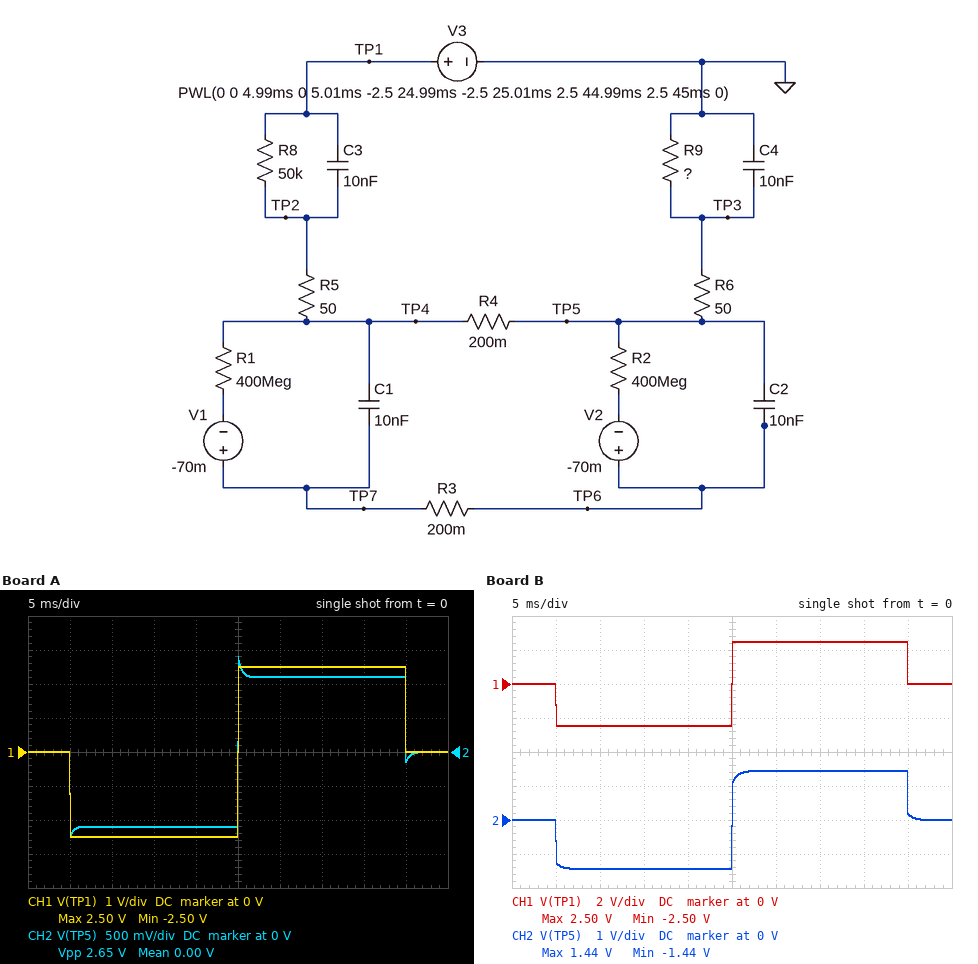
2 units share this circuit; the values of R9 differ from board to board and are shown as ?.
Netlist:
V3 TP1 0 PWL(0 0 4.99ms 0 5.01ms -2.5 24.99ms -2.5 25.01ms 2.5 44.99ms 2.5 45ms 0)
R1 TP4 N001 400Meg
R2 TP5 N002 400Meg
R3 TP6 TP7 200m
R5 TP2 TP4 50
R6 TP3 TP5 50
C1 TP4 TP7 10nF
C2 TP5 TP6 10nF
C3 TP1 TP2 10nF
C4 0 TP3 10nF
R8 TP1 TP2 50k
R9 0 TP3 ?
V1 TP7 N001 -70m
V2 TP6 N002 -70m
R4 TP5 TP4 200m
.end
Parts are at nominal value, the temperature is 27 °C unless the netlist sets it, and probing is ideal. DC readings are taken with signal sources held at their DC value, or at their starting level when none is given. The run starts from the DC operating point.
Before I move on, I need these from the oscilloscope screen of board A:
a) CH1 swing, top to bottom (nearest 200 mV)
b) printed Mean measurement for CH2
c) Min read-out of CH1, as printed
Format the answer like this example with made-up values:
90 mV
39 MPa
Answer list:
5.0 V
0.00 V
-2.50 V
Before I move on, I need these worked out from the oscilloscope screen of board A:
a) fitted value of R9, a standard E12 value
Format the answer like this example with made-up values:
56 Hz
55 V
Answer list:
39 kΩ
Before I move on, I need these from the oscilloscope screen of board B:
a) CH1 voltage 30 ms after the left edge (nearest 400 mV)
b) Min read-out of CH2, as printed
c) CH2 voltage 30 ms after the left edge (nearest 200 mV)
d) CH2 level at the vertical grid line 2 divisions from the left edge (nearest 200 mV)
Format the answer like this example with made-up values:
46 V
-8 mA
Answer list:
2.4 V
-1.44 V
1.4 V
-1.4 V
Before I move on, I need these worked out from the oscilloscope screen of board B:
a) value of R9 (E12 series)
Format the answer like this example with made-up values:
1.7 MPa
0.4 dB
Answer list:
68 kΩ
